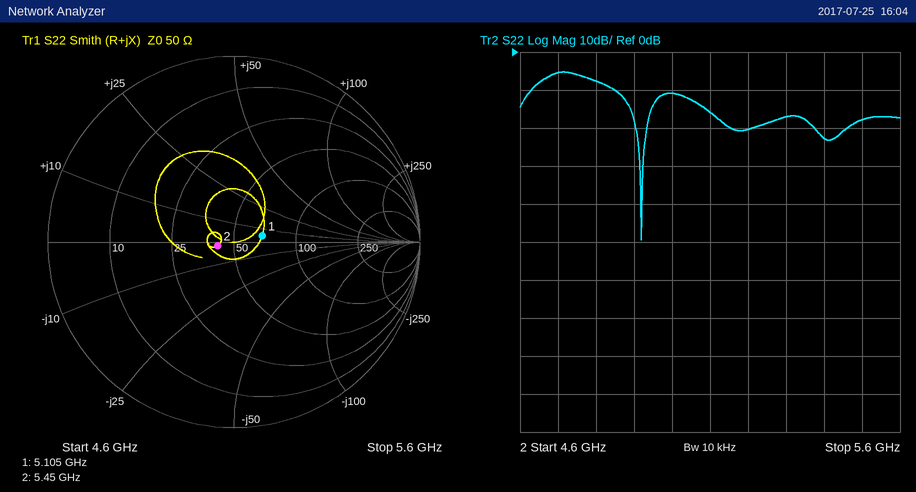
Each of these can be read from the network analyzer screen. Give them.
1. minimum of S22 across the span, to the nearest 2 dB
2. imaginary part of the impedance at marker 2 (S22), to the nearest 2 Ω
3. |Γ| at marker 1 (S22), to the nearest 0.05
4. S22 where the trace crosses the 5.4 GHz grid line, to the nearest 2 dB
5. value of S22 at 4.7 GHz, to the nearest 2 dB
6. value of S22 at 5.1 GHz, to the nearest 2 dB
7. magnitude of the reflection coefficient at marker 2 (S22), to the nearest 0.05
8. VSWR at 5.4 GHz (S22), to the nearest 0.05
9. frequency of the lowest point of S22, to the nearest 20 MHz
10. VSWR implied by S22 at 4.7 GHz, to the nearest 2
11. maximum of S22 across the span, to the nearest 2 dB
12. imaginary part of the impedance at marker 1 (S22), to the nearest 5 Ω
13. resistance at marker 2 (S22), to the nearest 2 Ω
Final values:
-50 dB
-2 Ω
0.15
-22 dB
-6 dB
-16 dB
0.10
1.15
4.92 GHz
4
-6 dB
+5 Ω
42 Ω
